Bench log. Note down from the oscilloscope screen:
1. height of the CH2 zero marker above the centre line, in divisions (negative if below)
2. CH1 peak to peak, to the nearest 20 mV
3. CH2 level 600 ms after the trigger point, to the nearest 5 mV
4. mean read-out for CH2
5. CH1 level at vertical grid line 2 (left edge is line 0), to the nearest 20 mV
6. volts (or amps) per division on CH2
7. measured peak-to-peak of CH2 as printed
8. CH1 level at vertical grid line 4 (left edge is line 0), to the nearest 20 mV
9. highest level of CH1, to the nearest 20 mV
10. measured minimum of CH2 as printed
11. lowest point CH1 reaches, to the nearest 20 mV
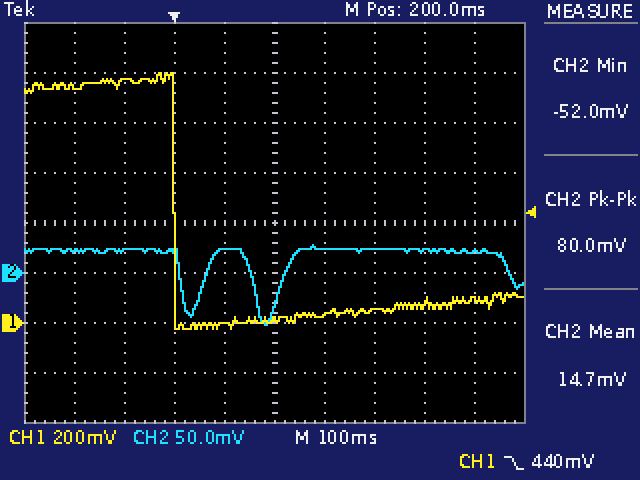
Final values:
-1.0 div
1.02 V
20 mV
14.7 mV
980 mV
50 mV
80.0 mV
0 mV
1.00 V
-52.0 mV
-20 mV
